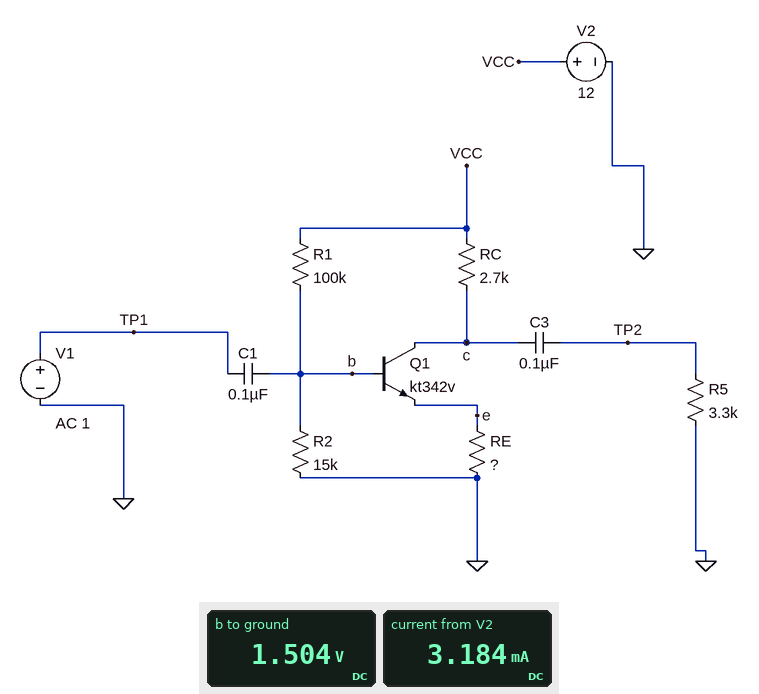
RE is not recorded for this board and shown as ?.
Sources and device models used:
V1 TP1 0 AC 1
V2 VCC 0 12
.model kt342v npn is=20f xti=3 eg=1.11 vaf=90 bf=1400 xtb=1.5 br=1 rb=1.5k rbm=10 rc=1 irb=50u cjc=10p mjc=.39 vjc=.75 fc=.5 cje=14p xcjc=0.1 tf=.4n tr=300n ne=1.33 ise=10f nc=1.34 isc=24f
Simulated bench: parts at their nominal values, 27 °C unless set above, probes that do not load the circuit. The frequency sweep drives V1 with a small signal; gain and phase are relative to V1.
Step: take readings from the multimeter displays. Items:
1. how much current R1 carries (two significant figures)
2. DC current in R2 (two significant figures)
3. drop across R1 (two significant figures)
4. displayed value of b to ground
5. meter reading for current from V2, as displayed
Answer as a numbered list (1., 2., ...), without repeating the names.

1. 100 µA
2. 100 µA
3. 10 V
4. 1.504 V
5. 3.184 mA
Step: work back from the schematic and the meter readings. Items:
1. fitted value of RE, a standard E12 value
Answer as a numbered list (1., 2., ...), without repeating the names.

1. 270 Ω
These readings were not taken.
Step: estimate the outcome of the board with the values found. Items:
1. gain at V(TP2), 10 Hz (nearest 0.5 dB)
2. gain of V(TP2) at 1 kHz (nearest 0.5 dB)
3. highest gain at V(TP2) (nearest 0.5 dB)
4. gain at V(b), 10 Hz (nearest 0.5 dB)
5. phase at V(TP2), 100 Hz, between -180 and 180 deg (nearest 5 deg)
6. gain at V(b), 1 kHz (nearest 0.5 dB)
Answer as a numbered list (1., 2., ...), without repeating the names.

1. -36.5 dB
2. 14.0 dB
3. 14.5 dB
4. -22.5 dB
5. -60 deg
6. 0 dB
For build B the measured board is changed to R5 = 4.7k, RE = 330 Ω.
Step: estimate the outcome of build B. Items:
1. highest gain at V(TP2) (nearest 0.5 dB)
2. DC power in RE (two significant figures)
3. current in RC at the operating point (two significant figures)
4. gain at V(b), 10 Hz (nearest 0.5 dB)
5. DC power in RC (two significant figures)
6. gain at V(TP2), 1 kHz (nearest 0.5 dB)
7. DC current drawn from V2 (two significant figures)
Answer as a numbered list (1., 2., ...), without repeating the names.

1. 14.0 dB
2. 2.2 mW
3. 2.6 mA
4. -22.0 dB
5. 18 mW
6. 13.5 dB
7. 2.7 mA
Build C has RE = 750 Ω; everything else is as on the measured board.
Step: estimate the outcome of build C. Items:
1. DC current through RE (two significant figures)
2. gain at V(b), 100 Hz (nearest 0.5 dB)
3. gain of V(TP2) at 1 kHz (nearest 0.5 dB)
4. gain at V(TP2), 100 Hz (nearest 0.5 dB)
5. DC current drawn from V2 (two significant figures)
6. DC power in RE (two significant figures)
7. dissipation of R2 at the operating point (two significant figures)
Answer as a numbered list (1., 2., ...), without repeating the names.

1. 1.2 mA
2. -4.0 dB
3. 5.5 dB
4. -7.5 dB
5. 1.3 mA
6. 1.1 mW
7. 160 µW
